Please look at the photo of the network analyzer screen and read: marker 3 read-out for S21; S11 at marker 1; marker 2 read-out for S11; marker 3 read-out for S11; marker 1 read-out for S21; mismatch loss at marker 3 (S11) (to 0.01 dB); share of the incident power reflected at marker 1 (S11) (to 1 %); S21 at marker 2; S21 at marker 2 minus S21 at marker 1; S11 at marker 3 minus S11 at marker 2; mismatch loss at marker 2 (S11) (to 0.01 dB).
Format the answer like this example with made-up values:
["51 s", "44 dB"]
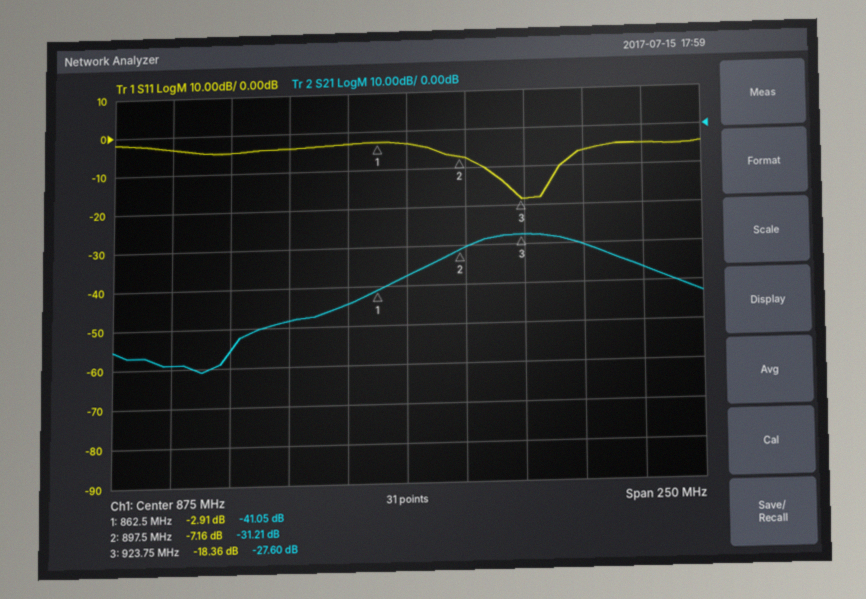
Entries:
["-27.60 dB", "-2.91 dB", "-7.16 dB", "-18.36 dB", "-41.05 dB", "0.06 dB", "51 %", "-31.21 dB", "9.84 dB", "-11.20 dB", "0.93 dB"]
